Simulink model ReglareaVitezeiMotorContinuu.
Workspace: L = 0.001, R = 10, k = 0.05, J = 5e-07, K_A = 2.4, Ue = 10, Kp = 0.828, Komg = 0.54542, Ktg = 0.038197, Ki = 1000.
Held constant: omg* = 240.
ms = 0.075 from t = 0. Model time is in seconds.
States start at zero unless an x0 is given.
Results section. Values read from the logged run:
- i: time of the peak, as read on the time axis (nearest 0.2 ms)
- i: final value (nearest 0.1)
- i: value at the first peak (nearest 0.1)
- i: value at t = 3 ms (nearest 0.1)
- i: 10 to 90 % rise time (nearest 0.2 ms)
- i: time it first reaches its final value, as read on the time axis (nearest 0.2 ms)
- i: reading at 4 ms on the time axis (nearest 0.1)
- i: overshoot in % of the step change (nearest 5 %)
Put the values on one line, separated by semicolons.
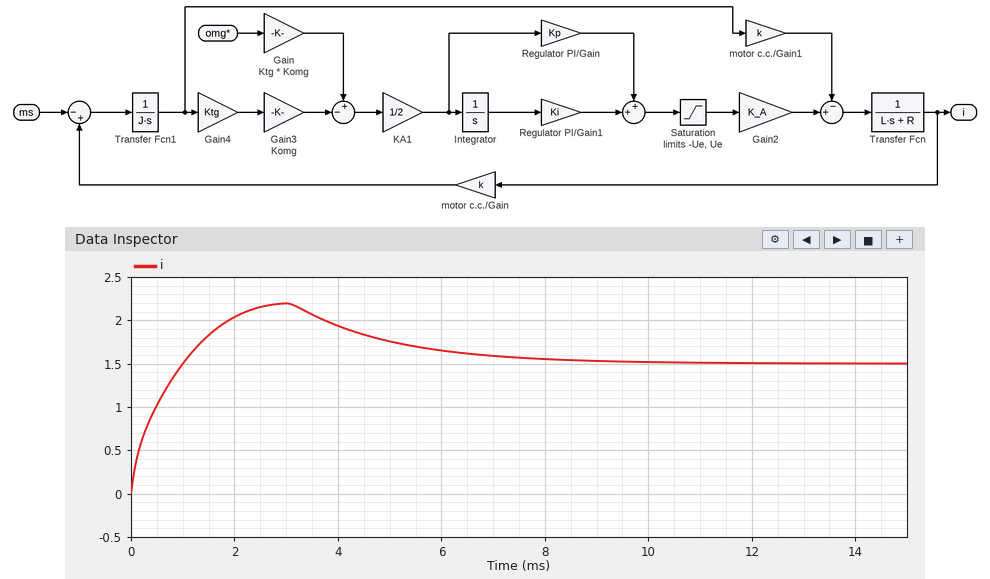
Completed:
3.0 ms; 1.5; 2.2; 2.2; 0.8 ms; 1.0 ms; 1.9; 45 %
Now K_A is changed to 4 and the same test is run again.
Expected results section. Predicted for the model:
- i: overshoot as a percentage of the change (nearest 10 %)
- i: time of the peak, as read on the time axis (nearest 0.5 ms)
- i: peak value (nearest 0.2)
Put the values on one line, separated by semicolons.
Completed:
60 %; 2.0 ms; 2.4
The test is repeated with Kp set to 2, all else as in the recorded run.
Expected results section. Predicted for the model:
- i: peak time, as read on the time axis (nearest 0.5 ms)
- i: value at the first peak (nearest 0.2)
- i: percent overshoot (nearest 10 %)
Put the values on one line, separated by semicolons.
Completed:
2.0 ms; 2.0; 30 %
